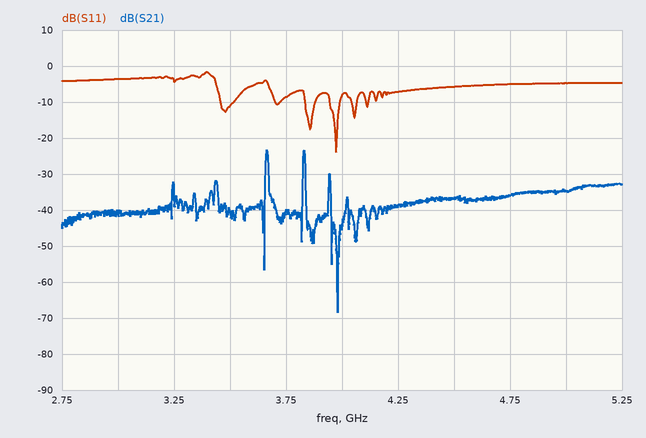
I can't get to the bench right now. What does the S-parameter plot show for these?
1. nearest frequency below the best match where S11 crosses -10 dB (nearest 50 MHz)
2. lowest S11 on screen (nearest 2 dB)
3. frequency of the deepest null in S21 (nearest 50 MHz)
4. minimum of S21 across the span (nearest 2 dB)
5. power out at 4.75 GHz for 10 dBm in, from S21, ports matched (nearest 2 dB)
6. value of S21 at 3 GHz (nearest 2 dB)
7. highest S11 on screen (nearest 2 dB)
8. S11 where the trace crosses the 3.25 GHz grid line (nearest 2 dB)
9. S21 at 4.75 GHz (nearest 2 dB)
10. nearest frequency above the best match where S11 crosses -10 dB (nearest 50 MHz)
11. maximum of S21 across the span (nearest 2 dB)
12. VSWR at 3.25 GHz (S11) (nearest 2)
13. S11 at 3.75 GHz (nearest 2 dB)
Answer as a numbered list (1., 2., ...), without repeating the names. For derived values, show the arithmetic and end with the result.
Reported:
1. 3.95 GHz
2. -24 dB
3. 4.00 GHz
4. -68 dB
5. 10 dBm + (-36 dB) = -26 dBm
6. -40 dB
7. -2 dB
8. -4 dB
9. -36 dB
10. 4.00 GHz
11. -24 dB
12. |Γ| = 10^(-4/20) = 0.6310; VSWR = (1 + 0.6310)/(1 − 0.6310) ≈ 4
13. -8 dB
